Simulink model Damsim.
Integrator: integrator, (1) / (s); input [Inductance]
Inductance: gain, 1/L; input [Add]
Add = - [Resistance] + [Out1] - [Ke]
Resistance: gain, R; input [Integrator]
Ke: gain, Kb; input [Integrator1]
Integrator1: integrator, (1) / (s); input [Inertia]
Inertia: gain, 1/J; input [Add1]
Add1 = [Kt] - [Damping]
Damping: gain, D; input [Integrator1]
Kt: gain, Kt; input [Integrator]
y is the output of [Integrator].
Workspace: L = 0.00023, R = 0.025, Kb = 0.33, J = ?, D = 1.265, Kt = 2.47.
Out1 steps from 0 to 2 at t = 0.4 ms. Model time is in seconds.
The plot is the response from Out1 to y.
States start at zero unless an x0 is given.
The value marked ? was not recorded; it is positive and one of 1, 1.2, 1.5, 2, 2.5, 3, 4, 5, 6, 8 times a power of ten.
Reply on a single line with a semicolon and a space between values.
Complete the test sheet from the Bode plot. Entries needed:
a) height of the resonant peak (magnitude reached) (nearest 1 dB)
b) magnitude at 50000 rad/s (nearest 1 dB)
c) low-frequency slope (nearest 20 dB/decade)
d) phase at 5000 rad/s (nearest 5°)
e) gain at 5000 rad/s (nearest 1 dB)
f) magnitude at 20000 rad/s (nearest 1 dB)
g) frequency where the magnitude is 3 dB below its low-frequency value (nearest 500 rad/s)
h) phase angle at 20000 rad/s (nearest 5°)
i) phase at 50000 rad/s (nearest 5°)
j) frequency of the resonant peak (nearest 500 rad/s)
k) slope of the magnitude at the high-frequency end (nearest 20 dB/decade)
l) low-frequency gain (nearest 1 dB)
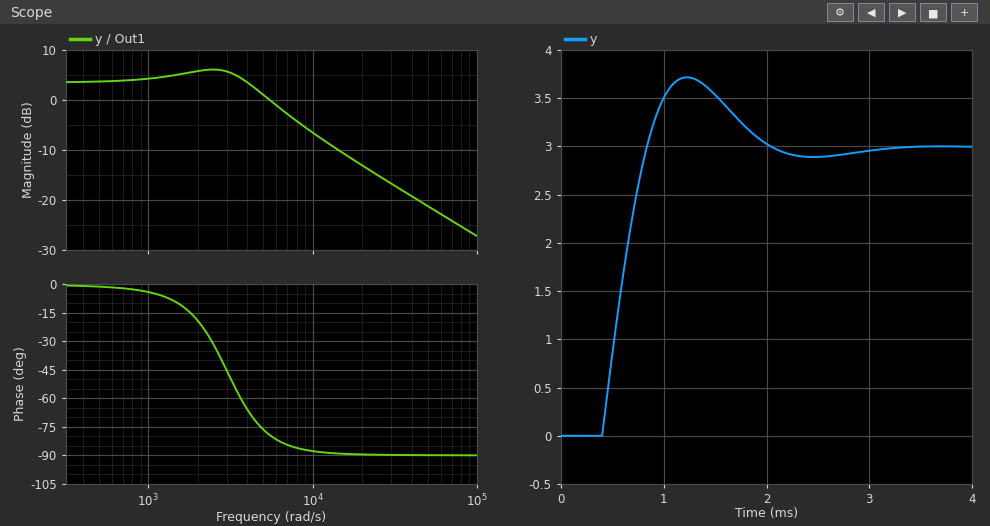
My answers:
6 dB; -21 dB; 0 dB/decade; -75°; 1 dB; -13 dB; 5000 rad/s; -90°; -90°; 2500 rad/s; -20 dB/decade; 4 dB
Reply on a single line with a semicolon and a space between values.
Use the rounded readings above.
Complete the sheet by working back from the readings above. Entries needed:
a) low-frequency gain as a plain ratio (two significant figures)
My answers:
1.6
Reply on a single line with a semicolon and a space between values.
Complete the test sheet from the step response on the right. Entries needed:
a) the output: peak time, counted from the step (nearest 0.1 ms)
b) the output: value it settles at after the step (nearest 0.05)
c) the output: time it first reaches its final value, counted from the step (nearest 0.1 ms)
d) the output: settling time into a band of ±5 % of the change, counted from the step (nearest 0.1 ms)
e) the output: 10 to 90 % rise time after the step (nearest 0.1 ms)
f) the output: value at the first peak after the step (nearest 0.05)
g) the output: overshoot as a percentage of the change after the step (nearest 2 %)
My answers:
0.8 ms; 3.00; 0.4 ms; 1.5 ms; 0.3 ms; 3.70; 24 %
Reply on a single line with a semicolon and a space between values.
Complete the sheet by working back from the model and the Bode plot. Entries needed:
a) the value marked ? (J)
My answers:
0.0004
